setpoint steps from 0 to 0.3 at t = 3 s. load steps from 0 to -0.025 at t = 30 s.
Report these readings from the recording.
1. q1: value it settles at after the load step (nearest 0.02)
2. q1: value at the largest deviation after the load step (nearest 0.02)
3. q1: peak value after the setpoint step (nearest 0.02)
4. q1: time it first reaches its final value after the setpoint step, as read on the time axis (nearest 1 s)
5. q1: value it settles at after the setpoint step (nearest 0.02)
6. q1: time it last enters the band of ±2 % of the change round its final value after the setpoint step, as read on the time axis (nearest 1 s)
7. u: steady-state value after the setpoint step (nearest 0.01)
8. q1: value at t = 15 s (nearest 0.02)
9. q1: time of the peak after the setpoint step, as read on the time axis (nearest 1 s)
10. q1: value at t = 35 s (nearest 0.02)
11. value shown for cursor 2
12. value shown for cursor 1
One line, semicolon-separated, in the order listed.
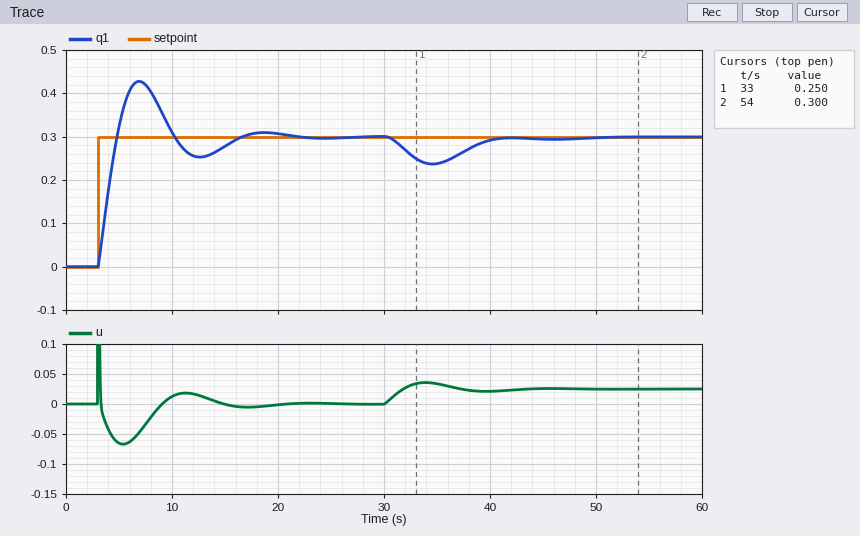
0.30; 0.24; 0.42; 5 s; 0.30; 20 s; 0.00; 0.28; 7 s; 0.24; 0.300; 0.250
